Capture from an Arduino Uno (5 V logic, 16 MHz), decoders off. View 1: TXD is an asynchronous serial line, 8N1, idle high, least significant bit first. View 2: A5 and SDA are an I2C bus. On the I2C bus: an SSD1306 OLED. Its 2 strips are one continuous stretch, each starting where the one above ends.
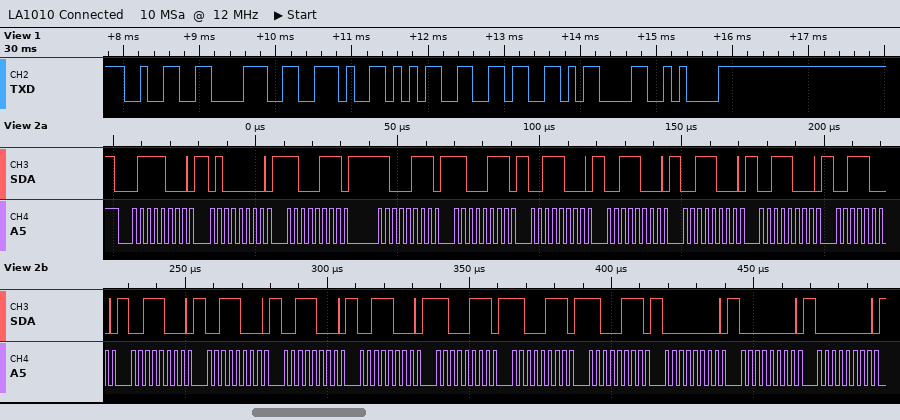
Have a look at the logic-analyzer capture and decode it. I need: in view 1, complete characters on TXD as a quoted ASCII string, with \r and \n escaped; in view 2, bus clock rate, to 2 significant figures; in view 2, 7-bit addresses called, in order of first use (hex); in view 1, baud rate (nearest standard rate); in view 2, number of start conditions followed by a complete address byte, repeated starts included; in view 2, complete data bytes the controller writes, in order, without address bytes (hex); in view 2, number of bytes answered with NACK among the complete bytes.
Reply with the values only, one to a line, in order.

"28.56\r\n"
400 kHz
0x3C
9600 baud
1
40 C7 C7 C7 38 38 38 38 38 38 38 38 38 C7 C7 C7 00 00 00
0
